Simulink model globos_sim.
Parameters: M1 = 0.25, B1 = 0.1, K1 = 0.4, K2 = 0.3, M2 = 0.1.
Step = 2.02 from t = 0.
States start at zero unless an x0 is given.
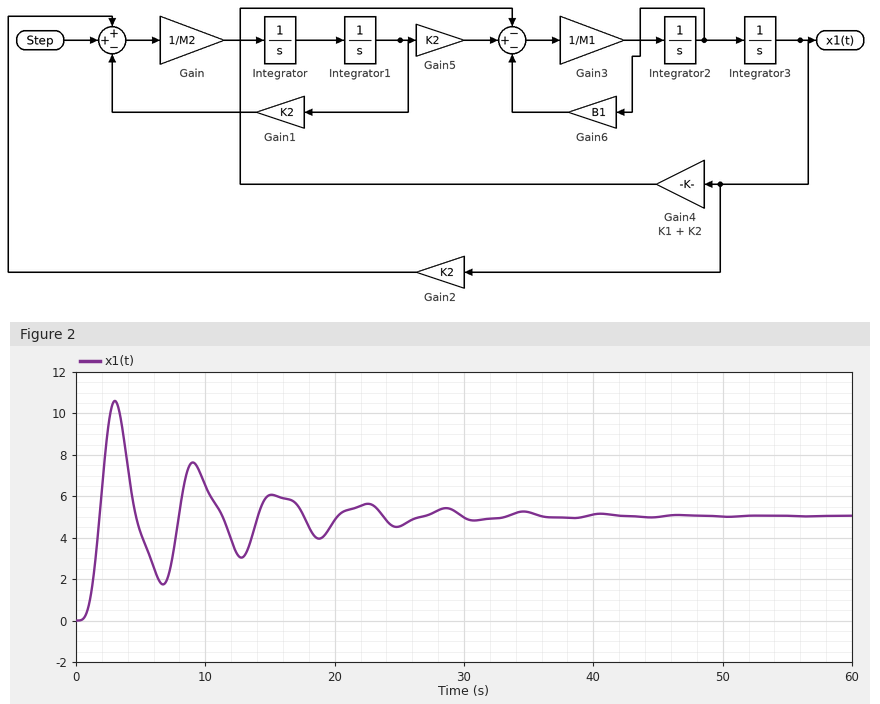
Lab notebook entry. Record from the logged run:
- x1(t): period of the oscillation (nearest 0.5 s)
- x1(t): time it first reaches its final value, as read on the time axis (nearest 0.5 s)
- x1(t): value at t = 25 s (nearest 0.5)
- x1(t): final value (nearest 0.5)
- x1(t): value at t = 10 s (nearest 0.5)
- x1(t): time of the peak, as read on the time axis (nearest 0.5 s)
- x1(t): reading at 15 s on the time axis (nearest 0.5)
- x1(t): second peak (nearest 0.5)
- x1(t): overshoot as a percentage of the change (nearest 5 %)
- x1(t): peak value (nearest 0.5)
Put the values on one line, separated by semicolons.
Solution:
6.0 s; 2.0 s; 4.5; 5.0; 6.5; 3.0 s; 6.0; 7.5; 110 %; 10.5
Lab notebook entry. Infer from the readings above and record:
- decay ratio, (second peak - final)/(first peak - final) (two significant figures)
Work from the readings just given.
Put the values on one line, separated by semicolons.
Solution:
0.45
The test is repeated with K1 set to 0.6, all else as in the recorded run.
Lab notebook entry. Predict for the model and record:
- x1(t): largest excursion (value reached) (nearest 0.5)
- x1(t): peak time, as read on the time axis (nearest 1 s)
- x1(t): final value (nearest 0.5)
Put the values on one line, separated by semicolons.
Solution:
8.0; 3 s; 3.5
